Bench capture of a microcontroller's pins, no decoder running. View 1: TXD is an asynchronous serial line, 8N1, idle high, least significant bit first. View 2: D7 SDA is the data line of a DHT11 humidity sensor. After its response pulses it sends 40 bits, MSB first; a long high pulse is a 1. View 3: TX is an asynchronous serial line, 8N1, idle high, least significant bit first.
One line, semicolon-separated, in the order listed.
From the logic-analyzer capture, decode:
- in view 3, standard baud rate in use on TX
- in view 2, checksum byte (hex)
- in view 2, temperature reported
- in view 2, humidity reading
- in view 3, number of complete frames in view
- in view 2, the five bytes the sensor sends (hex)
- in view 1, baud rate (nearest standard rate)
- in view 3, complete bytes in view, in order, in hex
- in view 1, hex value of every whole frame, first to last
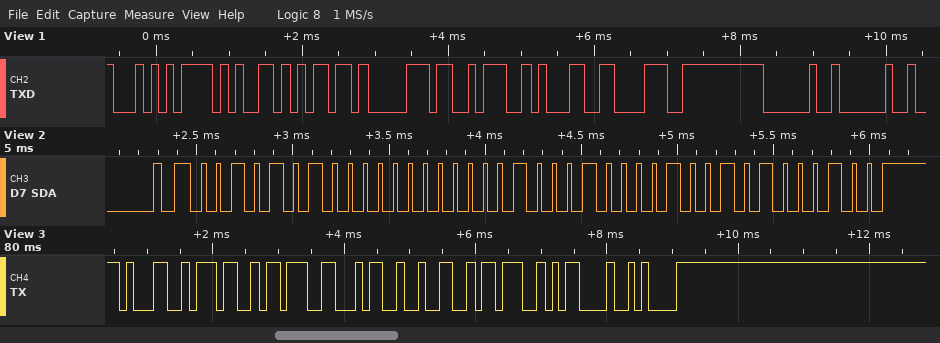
9600 baud; 0x44; 17.9 °C; 42 %; 8; 2A 00 11 09 44; 9600 baud; 31 37 3B 34 32 3B 0D 0A; 54 65 6D 70 3A 31 38 20 20
